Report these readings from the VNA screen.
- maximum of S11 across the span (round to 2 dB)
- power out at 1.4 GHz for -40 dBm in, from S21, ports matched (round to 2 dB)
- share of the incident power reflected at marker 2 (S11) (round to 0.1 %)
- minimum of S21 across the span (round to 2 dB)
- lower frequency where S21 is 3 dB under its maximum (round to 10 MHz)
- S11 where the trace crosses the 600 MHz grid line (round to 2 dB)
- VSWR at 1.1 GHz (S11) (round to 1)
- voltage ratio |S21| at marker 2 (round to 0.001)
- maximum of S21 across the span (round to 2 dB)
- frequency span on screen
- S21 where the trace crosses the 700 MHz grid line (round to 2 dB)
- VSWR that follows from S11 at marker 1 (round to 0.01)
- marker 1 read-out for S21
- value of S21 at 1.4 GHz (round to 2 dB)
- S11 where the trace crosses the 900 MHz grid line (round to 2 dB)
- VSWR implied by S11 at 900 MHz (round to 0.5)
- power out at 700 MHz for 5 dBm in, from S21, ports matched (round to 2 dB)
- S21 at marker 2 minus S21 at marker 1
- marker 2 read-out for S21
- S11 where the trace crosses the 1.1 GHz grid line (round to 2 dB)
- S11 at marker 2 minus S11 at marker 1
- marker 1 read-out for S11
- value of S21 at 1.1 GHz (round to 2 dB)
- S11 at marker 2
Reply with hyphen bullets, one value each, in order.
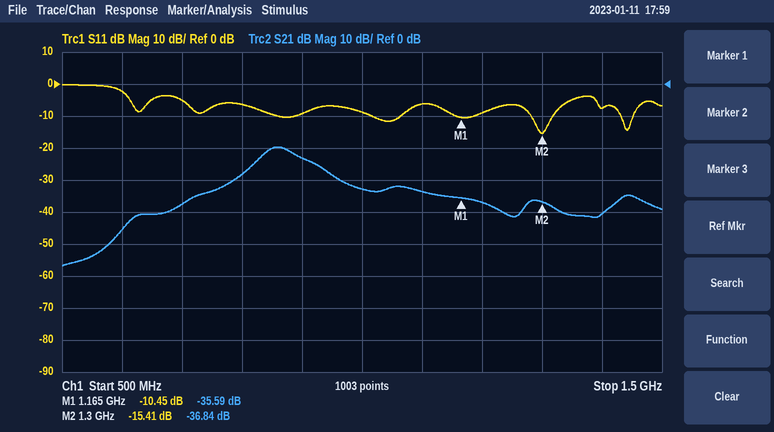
- 0 dB
- -80 dBm
- 2.9 %
- -56 dB
- 830 MHz
- -2 dB
- 3
- 0.014
- -20 dB
- 1 GHz
- -38 dB
- 1.86
- -35.59 dB
- -40 dB
- -10 dB
- 2.0
- -32 dBm
- -1.25 dB
- -36.84 dB
- -6 dB
- -4.96 dB
- -10.45 dB
- -34 dB
- -15.41 dB
